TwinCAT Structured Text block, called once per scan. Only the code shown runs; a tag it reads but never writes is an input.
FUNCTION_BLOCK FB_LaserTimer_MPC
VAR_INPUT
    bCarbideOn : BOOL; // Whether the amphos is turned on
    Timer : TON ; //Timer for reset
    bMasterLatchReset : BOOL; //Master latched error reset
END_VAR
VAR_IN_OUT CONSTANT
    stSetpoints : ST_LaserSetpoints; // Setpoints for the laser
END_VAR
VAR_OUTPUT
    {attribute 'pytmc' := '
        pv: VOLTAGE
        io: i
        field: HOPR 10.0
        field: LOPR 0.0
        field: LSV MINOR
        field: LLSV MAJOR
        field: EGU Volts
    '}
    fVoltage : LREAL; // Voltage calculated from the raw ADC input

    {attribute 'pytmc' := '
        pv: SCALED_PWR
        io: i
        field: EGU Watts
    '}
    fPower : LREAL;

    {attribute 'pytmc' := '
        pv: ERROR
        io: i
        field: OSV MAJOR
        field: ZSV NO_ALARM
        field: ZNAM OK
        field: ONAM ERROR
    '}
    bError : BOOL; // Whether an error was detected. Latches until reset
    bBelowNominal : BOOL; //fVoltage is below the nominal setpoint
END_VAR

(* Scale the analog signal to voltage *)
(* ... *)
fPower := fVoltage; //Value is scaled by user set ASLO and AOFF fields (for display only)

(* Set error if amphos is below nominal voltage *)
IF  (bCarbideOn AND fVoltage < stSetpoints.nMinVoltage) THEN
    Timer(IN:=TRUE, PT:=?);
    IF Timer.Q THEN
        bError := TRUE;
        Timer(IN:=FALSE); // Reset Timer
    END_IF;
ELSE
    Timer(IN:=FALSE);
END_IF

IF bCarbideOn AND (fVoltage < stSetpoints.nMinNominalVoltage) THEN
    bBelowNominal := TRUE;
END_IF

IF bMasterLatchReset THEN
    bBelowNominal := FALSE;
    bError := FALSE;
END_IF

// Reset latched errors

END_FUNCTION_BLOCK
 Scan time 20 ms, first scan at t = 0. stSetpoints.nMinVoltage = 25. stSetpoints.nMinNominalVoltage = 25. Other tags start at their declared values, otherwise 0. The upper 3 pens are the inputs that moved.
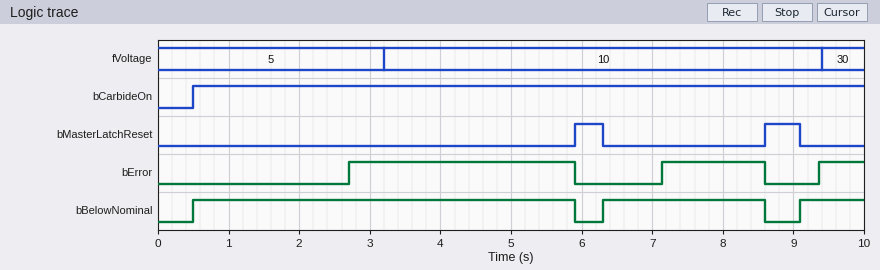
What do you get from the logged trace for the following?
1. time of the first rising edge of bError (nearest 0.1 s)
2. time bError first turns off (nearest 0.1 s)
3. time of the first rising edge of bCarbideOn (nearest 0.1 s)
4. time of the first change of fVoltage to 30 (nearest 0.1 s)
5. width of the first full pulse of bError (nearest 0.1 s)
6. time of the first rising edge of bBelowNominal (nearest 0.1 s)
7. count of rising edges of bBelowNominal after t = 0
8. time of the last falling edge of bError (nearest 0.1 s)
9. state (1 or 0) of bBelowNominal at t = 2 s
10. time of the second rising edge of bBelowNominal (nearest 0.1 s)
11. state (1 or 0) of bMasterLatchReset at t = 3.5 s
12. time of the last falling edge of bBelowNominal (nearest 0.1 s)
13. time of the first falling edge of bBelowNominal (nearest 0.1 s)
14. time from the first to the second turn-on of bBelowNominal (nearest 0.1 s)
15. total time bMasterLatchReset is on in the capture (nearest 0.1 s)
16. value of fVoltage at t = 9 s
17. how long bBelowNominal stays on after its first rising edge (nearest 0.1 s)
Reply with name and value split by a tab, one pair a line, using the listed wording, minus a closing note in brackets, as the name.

time of the first rising edge of bError	2.7 s
time bError first turns off	5.9 s
time of the first rising edge of bCarbideOn	0.5 s
time of the first change of fVoltage to 30	9.4 s
width of the first full pulse of bError	3.2 s
time of the first rising edge of bBelowNominal	0.5 s
count of rising edges of bBelowNominal after t = 0	3
time of the last falling edge of bError	8.6 s
state (1 or 0) of bBelowNominal at t = 2 s	1
time of the second rising edge of bBelowNominal	6.3 s
state (1 or 0) of bMasterLatchReset at t = 3.5 s	0
time of the last falling edge of bBelowNominal	8.6 s
time of the first falling edge of bBelowNominal	5.9 s
time from the first to the second turn-on of bBelowNominal	5.8 s
total time bMasterLatchReset is on in the capture	0.9 s
value of fVoltage at t = 9 s	10
how long bBelowNominal stays on after its first rising edge	5.4 s
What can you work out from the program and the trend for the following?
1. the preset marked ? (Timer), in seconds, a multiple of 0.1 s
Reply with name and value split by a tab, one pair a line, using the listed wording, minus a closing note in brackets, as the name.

the preset marked ? (Timer), in seconds, a multiple of 0.1 s	2.2 s
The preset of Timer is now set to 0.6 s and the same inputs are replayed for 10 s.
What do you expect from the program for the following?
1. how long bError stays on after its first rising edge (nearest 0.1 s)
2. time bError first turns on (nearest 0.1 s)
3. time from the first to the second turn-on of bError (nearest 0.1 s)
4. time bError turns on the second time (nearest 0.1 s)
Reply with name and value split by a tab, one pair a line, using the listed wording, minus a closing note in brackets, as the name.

how long bError stays on after its first rising edge	4.8 s
time bError first turns on	1.1 s
time from the first to the second turn-on of bError	5.6 s
time bError turns on the second time	6.7 s
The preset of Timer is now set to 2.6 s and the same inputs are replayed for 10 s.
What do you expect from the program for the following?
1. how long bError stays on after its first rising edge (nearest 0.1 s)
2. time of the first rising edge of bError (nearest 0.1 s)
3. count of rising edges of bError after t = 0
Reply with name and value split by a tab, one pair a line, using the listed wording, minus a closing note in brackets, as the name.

how long bError stays on after its first rising edge	2.8 s
time of the first rising edge of bError	3.1 s
count of rising edges of bError after t = 0	2
